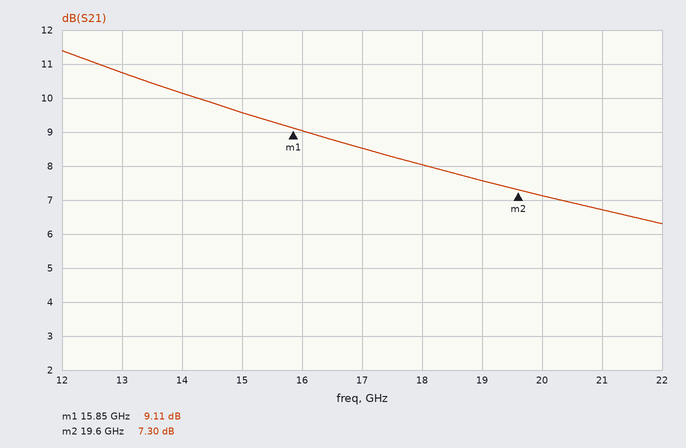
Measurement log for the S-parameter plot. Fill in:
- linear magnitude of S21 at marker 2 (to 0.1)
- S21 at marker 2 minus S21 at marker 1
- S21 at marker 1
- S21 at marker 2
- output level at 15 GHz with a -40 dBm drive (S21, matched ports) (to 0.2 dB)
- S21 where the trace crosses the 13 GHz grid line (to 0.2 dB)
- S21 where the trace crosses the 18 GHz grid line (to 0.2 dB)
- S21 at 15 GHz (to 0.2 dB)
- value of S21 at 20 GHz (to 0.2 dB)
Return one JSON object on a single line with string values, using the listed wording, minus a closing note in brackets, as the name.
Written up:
{"linear magnitude of S21 at marker 2": "2.3", "S21 at marker 2 minus S21 at marker 1": "-1.81 dB", "S21 at marker 1": "9.11 dB", "S21 at marker 2": "7.30 dB", "output level at 15 GHz with a -40 dBm drive (S21, matched ports)": "-30.4 dBm", "S21 where the trace crosses the 13 GHz grid line": "10.8 dB", "S21 where the trace crosses the 18 GHz grid line": "8.0 dB", "S21 at 15 GHz": "9.6 dB", "value of S21 at 20 GHz": "7.2 dB"}
